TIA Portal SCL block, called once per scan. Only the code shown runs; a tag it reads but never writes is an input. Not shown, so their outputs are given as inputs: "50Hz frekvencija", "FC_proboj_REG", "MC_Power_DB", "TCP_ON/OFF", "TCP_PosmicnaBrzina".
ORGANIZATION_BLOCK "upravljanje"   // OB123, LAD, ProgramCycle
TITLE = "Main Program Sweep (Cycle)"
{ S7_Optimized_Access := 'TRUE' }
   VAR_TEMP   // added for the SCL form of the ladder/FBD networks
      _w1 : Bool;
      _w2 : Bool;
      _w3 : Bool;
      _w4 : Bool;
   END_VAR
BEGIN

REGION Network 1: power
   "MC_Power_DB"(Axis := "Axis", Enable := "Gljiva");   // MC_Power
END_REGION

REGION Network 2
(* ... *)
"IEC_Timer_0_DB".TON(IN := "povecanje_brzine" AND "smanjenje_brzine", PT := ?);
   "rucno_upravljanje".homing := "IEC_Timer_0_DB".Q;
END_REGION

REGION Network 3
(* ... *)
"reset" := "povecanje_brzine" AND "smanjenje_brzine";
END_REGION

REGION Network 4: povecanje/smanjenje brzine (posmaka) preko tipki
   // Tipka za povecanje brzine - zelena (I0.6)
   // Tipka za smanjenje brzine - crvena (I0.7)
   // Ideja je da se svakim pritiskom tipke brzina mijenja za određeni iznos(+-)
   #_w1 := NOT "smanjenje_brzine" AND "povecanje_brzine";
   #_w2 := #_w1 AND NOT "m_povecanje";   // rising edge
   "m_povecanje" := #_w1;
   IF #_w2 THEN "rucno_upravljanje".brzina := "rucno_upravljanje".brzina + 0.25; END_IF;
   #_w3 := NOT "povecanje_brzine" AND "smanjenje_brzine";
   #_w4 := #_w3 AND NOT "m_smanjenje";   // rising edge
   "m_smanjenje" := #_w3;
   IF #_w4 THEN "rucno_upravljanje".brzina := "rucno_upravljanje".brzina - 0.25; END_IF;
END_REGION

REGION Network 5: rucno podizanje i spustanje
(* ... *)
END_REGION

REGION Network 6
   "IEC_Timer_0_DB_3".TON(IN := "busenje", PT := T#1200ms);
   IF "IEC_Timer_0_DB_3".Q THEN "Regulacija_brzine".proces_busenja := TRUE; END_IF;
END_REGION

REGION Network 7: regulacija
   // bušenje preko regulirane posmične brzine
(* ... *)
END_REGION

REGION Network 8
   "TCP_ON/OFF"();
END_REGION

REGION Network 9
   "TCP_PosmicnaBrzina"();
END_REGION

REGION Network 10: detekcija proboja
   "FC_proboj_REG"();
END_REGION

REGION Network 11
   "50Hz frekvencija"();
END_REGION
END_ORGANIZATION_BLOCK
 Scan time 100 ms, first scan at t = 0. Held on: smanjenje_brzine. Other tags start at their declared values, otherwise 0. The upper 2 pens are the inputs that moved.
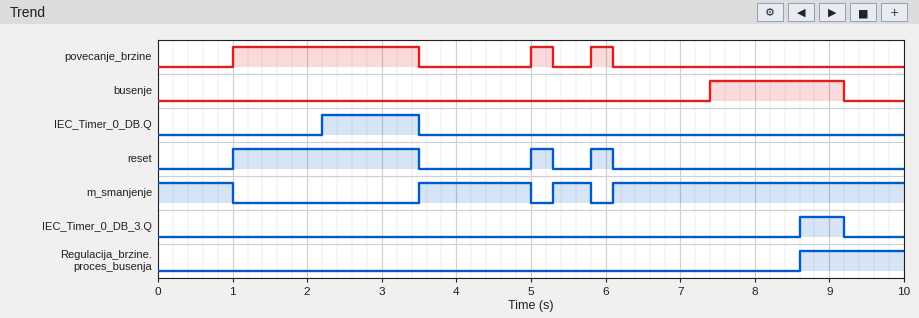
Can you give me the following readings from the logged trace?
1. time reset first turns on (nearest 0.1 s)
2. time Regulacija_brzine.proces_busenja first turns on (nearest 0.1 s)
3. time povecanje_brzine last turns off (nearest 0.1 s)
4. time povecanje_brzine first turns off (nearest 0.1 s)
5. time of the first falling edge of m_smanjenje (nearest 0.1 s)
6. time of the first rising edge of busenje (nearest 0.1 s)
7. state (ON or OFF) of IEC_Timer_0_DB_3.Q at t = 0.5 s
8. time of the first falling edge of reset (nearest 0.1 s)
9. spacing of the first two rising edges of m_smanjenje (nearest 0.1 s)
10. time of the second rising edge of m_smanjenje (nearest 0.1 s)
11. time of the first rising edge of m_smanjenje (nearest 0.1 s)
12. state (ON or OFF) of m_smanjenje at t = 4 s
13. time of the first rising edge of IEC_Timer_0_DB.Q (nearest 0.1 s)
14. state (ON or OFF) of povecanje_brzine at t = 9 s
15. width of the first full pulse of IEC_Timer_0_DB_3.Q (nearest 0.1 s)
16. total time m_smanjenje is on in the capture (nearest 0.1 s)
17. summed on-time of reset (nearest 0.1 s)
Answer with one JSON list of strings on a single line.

["1.0 s", "8.6 s", "6.1 s", "3.5 s", "1.0 s", "7.4 s", "OFF", "3.5 s", "1.8 s", "5.3 s", "3.5 s", "ON", "2.2 s", "OFF", "0.6 s", "6.9 s", "3.1 s"]
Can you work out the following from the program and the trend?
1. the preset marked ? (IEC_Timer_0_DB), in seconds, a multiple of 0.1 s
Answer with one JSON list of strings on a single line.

["1.2 s"]
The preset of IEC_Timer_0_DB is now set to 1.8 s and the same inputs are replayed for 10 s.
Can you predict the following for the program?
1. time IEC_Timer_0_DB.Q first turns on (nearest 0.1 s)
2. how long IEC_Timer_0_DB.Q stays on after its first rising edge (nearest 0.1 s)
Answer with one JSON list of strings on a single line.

["2.8 s", "0.7 s"]
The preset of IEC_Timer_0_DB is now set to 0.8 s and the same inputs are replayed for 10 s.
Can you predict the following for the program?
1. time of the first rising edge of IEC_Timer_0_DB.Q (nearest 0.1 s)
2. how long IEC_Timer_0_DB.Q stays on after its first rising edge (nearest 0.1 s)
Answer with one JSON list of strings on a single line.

["1.8 s", "1.7 s"]
